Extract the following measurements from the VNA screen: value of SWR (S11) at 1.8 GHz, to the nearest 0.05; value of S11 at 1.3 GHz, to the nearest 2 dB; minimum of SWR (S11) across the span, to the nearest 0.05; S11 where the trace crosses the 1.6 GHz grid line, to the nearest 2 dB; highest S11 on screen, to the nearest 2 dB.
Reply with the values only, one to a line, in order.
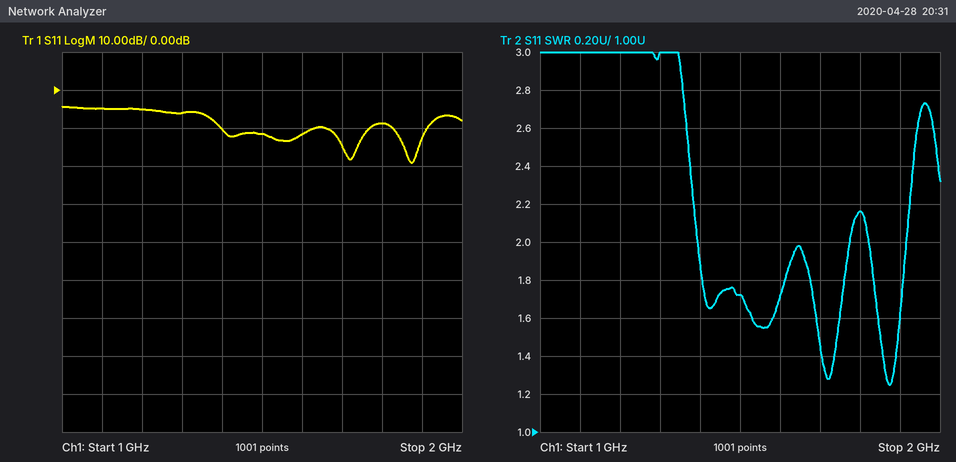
2.15
-6 dB
1.25
-12 dB
-4 dB
